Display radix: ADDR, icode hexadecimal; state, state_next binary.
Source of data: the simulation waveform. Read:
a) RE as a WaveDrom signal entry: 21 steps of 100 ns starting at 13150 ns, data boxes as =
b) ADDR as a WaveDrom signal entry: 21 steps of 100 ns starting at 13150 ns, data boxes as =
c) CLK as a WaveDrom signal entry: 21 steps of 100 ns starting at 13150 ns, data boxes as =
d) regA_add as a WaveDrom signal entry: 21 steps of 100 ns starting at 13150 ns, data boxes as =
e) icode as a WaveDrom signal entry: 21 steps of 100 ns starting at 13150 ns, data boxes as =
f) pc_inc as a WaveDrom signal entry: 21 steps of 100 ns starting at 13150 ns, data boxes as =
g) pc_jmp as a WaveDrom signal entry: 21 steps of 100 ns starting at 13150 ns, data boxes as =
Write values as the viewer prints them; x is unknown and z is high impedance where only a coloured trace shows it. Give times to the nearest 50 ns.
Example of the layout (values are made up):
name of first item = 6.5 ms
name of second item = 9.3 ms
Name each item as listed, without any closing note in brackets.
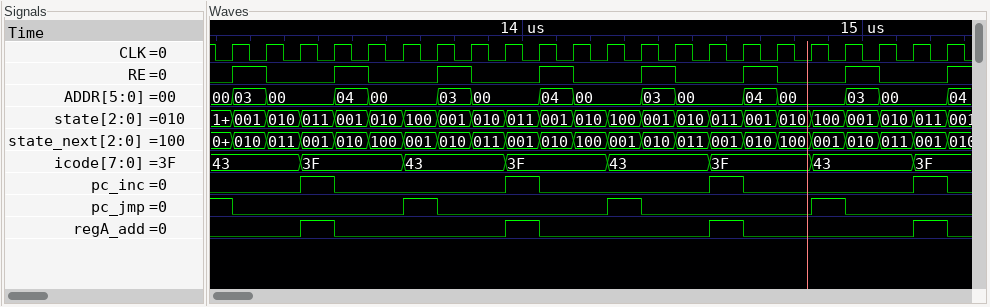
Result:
RE as a WaveDrom signal entry: 21 steps of 100 ns starting at 13150 ns, data boxes as = = {name: 'RE', wave: '10.10.10.10.10.10.10.'}
ADDR as a WaveDrom signal entry: 21 steps of 100 ns starting at 13150 ns, data boxes as = = {name: 'ADDR', wave: '==.==.==.==.==.==.==.', data: '03 00 04 00 03 00 04 00 03 00 04 00 03 00'}
CLK as a WaveDrom signal entry: 21 steps of 100 ns starting at 13150 ns, data boxes as = = {name: 'CLK', wave: 'p....................'}
regA_add as a WaveDrom signal entry: 21 steps of 100 ns starting at 13150 ns, data boxes as = = {name: 'regA_add', wave: '0.10....10....10....1'}
icode as a WaveDrom signal entry: 21 steps of 100 ns starting at 13150 ns, data boxes as = = {name: 'icode', wave: '=.=..=..=..=..=..=..=', data: '43 3F 43 3F 43 3F 43 3F'}
pc_inc as a WaveDrom signal entry: 21 steps of 100 ns starting at 13150 ns, data boxes as = = {name: 'pc_inc', wave: '0.10....10....10....1'}
pc_jmp as a WaveDrom signal entry: 21 steps of 100 ns starting at 13150 ns, data boxes as = = {name: 'pc_jmp', wave: '0....10....10....10..'}
